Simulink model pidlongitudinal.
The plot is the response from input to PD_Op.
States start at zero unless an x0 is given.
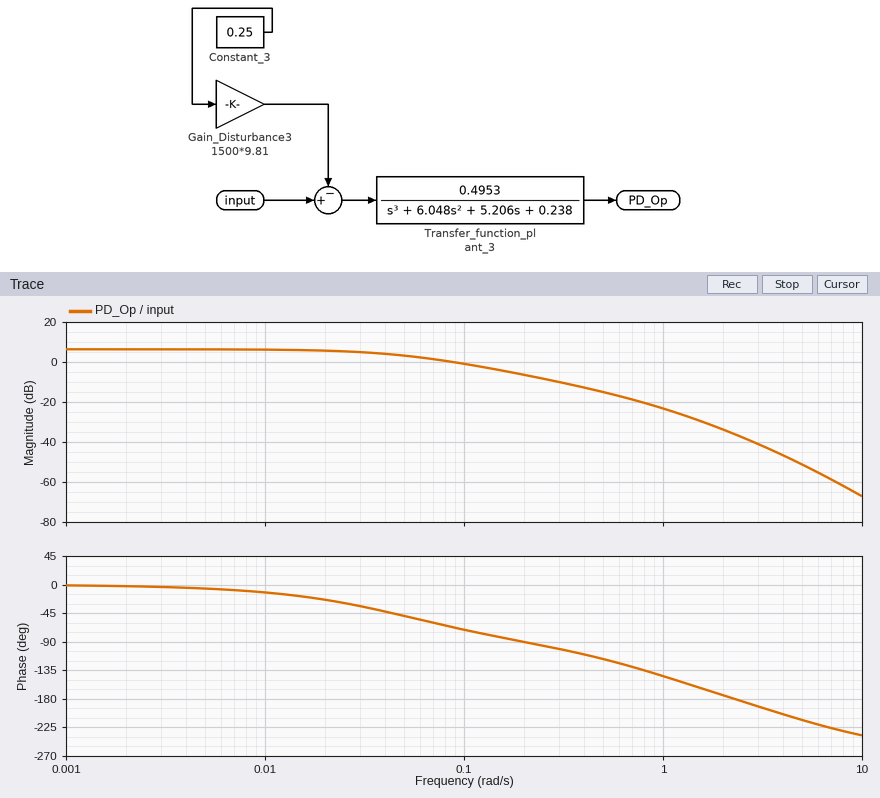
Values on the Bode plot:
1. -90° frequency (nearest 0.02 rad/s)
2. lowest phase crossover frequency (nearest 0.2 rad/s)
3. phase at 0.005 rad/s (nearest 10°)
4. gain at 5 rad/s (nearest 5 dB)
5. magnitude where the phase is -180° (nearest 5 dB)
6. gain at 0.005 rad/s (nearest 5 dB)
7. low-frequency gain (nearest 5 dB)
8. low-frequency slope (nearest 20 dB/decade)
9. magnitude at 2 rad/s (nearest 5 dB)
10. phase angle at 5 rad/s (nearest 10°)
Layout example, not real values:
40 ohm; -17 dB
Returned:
0.20 rad/s; 2.2 rad/s; -10°; -50 dB; -35 dB; 5 dB; 5 dB; 0 dB/decade; -35 dB; -210°
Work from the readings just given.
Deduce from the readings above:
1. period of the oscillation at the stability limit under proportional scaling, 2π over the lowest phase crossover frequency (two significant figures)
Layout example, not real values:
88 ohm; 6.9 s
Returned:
2.9 s
